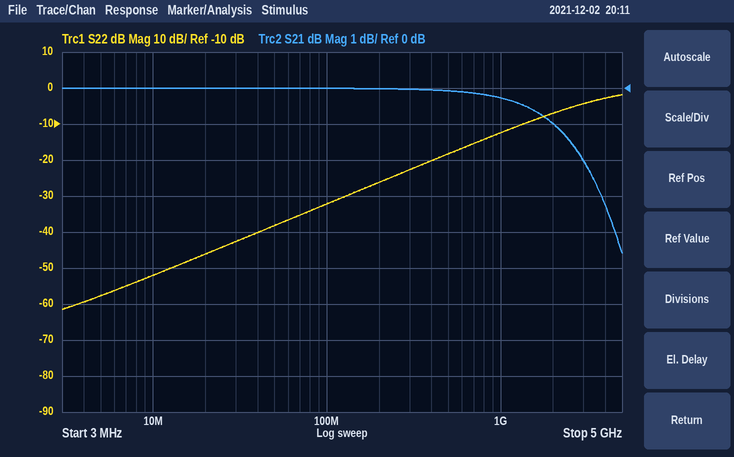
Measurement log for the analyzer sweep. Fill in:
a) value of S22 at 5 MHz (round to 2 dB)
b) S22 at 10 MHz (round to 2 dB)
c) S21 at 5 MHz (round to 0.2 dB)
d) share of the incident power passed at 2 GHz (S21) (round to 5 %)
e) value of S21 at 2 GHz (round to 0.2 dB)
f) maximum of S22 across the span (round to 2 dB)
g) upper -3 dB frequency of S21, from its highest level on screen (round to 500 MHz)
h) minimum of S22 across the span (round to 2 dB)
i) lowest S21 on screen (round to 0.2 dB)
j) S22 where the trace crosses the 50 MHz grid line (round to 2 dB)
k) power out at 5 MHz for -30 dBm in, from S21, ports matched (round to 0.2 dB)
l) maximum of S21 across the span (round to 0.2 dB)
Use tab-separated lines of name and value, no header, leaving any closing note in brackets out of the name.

value of S22 at 5 MHz	-58 dB
S22 at 10 MHz	-52 dB
S21 at 5 MHz	0.0 dB
share of the incident power passed at 2 GHz (S21)	80 %
value of S21 at 2 GHz	-1.0 dB
maximum of S22 across the span	-2 dB
upper -3 dB frequency of S21, from its highest level on screen	4.0 GHz
minimum of S22 across the span	-62 dB
lowest S21 on screen	-4.6 dB
S22 where the trace crosses the 50 MHz grid line	-38 dB
power out at 5 MHz for -30 dBm in, from S21, ports matched	-30.0 dBm
maximum of S21 across the span	0.0 dB
